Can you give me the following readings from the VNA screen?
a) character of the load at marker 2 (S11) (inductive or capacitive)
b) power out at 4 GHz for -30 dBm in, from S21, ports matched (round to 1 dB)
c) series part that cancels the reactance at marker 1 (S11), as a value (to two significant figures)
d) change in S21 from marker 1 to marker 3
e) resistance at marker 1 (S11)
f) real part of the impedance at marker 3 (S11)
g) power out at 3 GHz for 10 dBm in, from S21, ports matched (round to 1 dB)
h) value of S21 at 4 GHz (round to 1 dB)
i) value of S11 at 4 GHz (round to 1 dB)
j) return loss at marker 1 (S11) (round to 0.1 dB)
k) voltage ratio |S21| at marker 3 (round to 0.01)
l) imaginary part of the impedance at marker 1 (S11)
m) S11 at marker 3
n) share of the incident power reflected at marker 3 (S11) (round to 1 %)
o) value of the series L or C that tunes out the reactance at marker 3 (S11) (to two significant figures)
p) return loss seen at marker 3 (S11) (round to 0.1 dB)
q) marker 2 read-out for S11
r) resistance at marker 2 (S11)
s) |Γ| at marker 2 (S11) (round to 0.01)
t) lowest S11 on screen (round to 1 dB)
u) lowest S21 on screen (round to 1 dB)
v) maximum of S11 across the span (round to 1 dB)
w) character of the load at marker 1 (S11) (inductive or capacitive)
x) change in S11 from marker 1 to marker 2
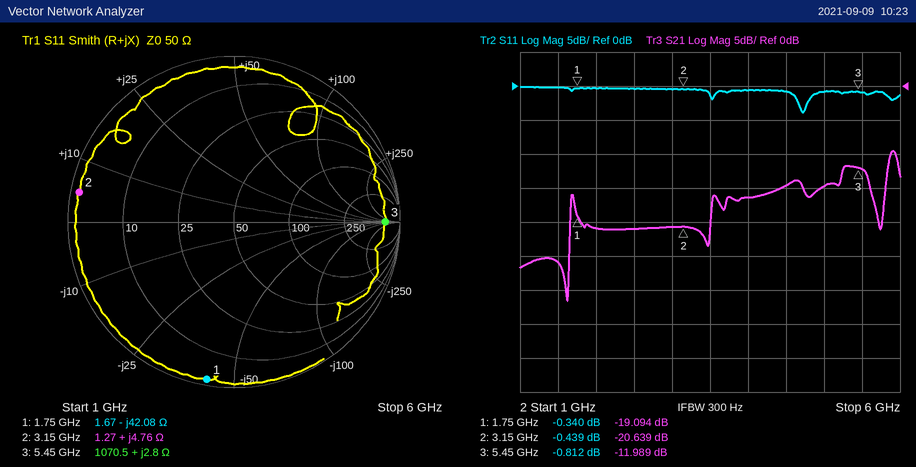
inductive
-46 dBm
3.8 nH
7.105 dB
1.67 Ω
1070.5 Ω
-11 dBm
-16 dB
-1 dB
0.3 dB
0.25
-42.08 Ω
-0.812 dB
83 %
10 pF
0.8 dB
-0.439 dB
1.27 Ω
0.95
-4 dB
-32 dB
0 dB
capacitive
-0.099 dB
